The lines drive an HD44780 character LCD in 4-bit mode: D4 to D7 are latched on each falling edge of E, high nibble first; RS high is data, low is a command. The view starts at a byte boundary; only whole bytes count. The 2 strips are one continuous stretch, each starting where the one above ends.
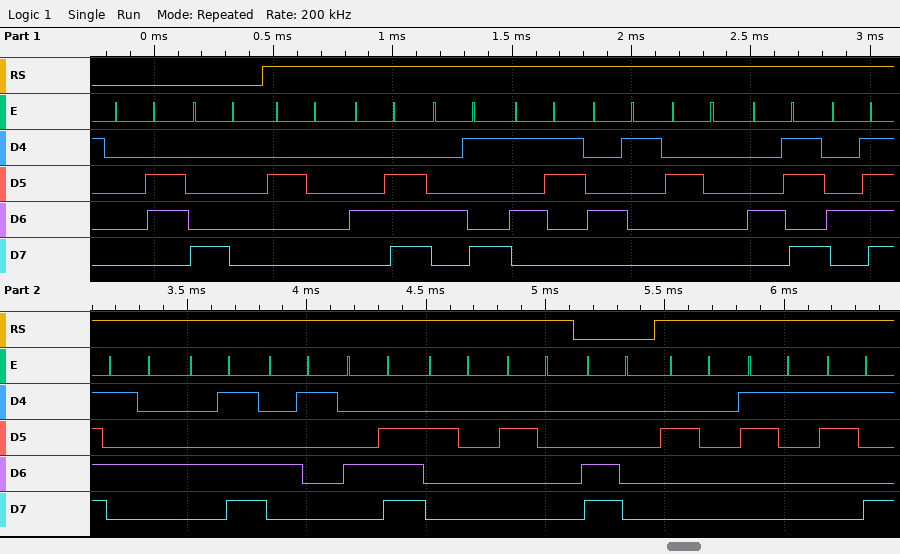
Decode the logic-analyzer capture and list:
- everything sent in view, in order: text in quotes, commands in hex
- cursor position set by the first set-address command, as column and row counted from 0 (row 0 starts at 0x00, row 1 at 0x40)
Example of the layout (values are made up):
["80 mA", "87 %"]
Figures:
["0x06 0x80 \" NISA KOTMAN  \" 0xC0 \" 19\"", "column 0, row 0"]
